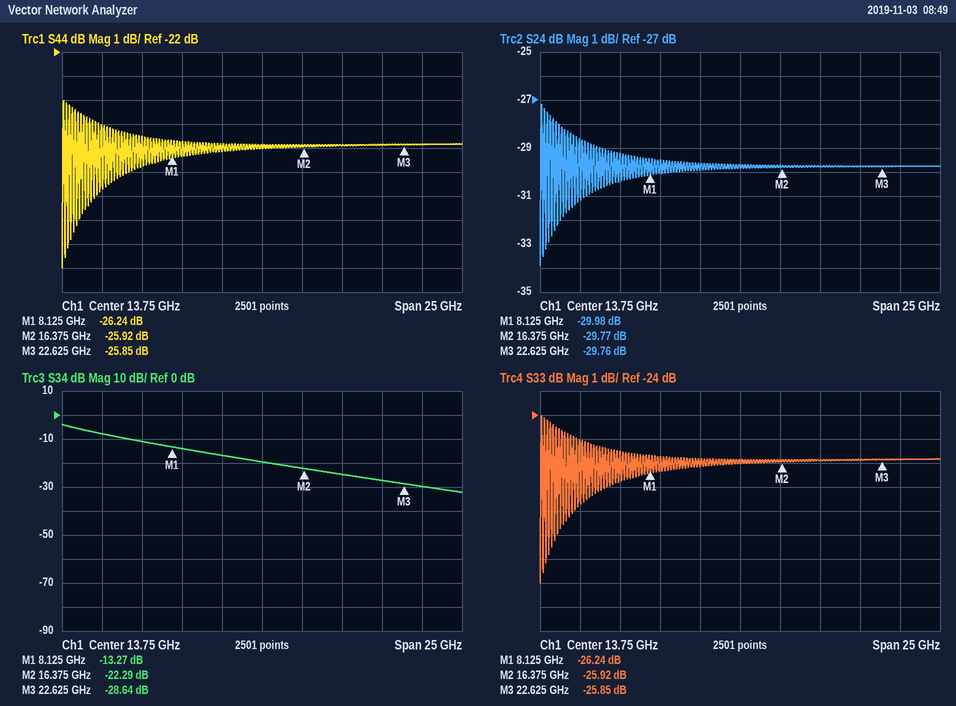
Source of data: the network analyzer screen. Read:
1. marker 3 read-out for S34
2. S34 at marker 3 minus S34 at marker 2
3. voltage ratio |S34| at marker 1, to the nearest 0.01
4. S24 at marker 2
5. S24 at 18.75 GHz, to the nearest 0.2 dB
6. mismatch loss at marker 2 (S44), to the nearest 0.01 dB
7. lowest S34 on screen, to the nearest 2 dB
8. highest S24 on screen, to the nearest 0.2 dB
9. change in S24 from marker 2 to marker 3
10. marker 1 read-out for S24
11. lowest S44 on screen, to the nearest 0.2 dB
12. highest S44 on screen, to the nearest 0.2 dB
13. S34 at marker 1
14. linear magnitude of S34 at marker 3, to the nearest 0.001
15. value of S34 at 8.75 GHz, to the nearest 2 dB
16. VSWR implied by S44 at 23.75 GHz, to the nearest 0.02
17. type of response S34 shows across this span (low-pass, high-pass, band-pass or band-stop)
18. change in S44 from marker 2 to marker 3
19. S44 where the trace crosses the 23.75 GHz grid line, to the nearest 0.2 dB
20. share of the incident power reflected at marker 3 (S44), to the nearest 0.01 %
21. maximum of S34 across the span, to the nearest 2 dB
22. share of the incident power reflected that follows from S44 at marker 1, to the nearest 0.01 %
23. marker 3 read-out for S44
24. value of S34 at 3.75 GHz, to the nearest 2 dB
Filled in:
-28.64 dB
-6.35 dB
0.22
-29.77 dB
-29.8 dB
0.01 dB
-32 dB
-27.2 dB
0.01 dB
-29.98 dB
-31.0 dB
-24.0 dB
-13.27 dB
0.037
-14 dB
1.10
low-pass
0.07 dB
-25.8 dB
0.26 %
-4 dB
0.24 %
-25.85 dB
-8 dB
